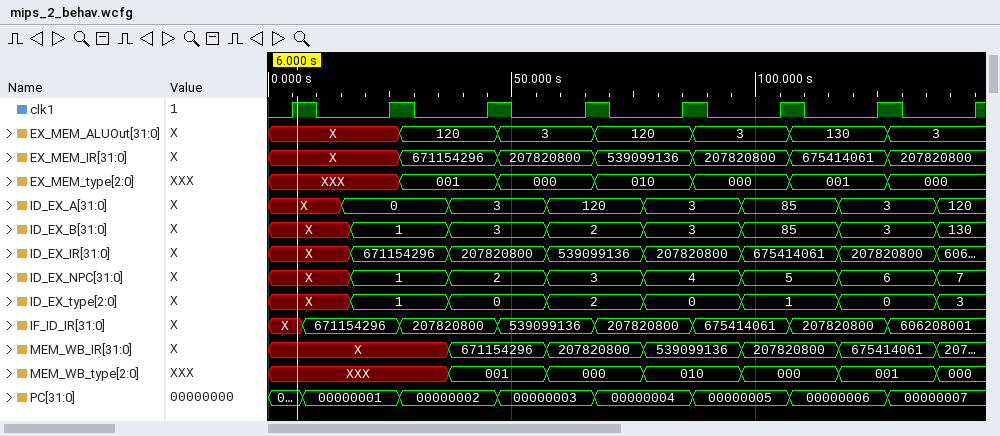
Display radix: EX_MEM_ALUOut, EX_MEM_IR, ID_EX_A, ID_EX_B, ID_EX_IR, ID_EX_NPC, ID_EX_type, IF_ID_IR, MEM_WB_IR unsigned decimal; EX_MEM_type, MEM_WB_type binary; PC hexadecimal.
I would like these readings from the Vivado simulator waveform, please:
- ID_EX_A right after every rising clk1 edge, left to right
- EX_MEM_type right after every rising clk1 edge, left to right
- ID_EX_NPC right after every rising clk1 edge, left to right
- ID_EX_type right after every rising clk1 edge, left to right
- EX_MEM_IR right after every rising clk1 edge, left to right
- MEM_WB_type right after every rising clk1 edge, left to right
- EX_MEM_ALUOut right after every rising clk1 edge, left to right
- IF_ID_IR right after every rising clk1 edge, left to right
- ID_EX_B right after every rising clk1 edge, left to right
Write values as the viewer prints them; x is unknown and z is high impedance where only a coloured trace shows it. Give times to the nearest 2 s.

X, 0, 3, 120, 3, 85, 3, 120
XXX, XXX, 001, 000, 010, 000, 001, 000
X, 1, 2, 3, 4, 5, 6, 7
X, 1, 0, 2, 0, 1, 0, 3
X, X, 671154296, 207820800, 539099136, 207820800, 675414061, 207820800
XXX, XXX, 001, 000, 010, 000, 001, 000
X, X, 120, 3, 120, 3, 130, 3
X, 671154296, 207820800, 539099136, 207820800, 675414061, 207820800, 606208001
X, 1, 3, 2, 3, 85, 3, 130
